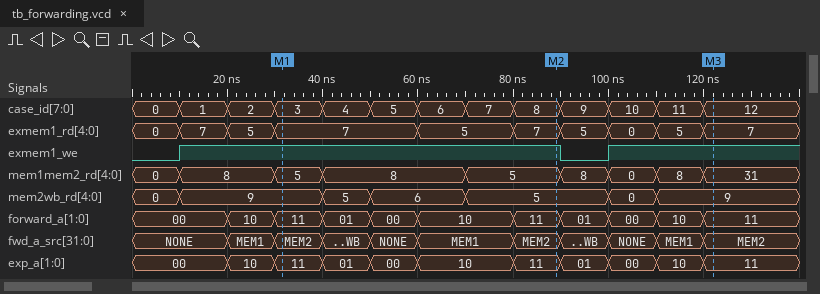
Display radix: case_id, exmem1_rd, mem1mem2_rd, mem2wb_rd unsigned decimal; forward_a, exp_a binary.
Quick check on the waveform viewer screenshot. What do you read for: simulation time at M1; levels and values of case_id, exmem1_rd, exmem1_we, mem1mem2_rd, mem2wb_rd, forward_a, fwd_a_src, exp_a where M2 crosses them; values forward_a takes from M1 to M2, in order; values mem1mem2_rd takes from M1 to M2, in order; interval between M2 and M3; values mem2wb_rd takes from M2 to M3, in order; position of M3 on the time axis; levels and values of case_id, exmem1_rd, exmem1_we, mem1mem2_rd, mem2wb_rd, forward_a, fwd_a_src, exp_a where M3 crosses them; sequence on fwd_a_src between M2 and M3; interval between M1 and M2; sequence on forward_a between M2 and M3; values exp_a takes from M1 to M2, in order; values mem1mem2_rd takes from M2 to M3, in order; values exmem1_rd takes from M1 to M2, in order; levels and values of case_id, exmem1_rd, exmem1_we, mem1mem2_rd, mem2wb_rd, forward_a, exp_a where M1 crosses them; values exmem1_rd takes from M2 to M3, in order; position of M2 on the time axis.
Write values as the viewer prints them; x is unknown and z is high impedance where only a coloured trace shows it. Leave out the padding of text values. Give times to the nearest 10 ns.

30 ns
case_id=8, exmem1_rd=7, exmem1_we=1, mem1mem2_rd=5, mem2wb_rd=5, forward_a=11, fwd_a_src=MEM2, exp_a=11
11, 01, 00, 10, 11
5, 8, 5
30 ns
5, 0, 9
120 ns
case_id=12, exmem1_rd=7, exmem1_we=1, mem1mem2_rd=31, mem2wb_rd=9, forward_a=11, fwd_a_src=MEM2, exp_a=11
MEM2, WB, NONE, MEM1, MEM2
60 ns
11, 01, 00, 10, 11
11, 01, 00, 10, 11
5, 8, 0, 8, 31
7, 5, 7
case_id=3, exmem1_rd=7, exmem1_we=1, mem1mem2_rd=5, mem2wb_rd=9, forward_a=11, exp_a=11
7, 5, 0, 5, 7
90 ns
